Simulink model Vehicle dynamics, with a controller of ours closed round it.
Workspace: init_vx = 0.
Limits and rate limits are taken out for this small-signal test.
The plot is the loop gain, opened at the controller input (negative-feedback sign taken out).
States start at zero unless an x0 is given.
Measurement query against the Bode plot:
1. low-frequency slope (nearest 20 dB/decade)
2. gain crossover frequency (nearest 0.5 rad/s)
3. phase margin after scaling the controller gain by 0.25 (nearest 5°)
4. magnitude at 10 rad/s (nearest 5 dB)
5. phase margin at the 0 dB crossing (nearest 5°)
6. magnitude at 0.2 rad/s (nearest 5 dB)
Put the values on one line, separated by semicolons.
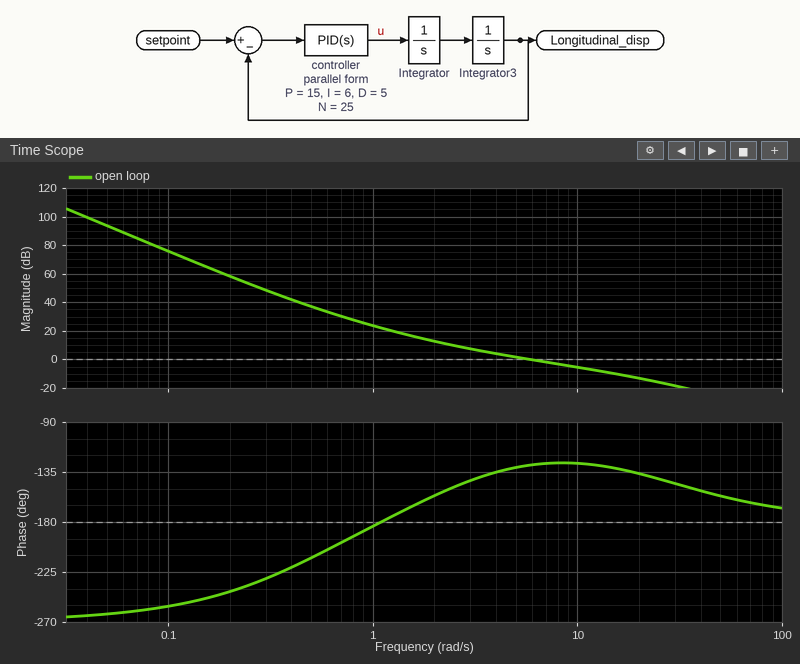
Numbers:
-60 dB/decade; 6.0 rad/s; 25°; -5 dB; 50°; 60 dB
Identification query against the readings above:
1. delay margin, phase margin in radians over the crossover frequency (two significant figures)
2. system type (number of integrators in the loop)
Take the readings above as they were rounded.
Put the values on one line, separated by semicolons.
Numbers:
0.15 s; 3
